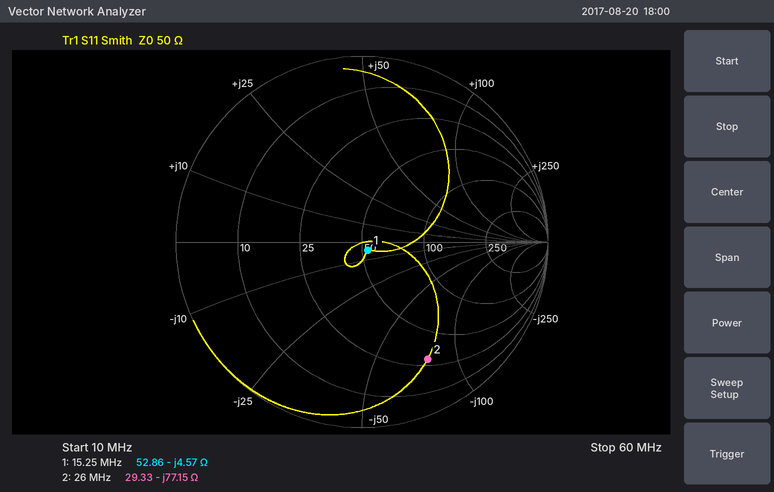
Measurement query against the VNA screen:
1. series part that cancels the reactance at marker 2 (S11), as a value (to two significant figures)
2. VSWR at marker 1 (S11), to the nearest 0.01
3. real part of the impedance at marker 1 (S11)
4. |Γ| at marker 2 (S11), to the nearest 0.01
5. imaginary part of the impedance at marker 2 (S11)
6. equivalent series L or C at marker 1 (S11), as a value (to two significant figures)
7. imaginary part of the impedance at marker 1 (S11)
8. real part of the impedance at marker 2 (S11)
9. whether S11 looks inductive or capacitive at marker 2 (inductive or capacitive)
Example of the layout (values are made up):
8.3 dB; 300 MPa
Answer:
470 nH; 1.11; 52.86 Ω; 0.72; -77.15 Ω; 2.3 nF; -4.57 Ω; 29.33 Ω; capacitive
